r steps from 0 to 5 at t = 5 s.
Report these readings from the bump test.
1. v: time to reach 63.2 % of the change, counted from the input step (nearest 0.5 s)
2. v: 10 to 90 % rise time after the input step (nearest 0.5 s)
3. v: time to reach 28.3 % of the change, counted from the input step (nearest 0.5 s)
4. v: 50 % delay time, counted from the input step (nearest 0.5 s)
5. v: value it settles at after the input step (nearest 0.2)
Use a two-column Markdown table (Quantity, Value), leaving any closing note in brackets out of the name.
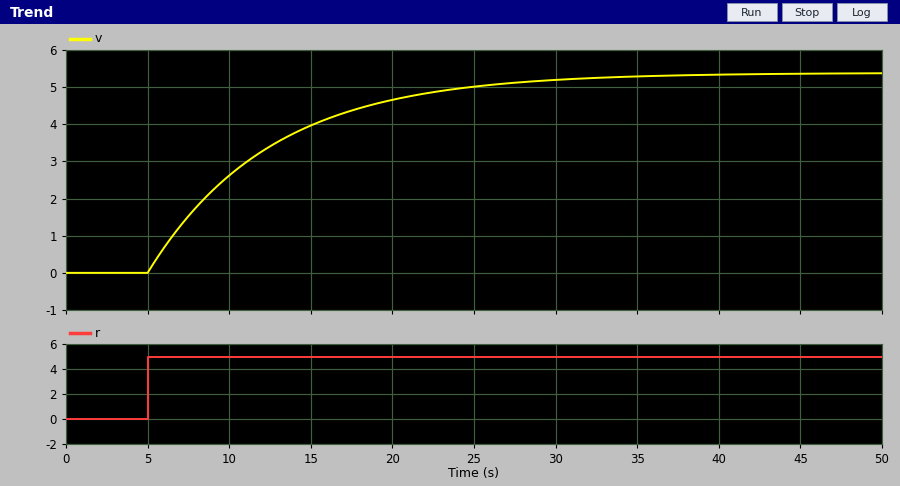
| Quantity | Value |
|---|---|
| v: time to reach 63.2 % of the change, counted from the input step | 7.5 s |
| v: 10 to 90 % rise time after the input step | 16.5 s |
| v: time to reach 28.3 % of the change, counted from the input step | 2.5 s |
| v: 50 % delay time, counted from the input step | 5.0 s |
| v: value it settles at after the input step | 5.4 |
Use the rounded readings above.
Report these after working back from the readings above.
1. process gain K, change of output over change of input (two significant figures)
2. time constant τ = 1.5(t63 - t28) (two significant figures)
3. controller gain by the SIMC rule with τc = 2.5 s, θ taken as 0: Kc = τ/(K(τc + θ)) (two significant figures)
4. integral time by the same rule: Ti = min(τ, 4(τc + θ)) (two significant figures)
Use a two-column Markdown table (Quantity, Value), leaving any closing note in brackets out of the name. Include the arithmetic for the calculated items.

| Quantity | Value |
|---|---|
| process gain K, change of output over change of input | (5.4 - 0) / 5 = 1.1 |
| time constant τ = 1.5(t63 - t28) | 1.5 × (7.5 - 2.5) = 7.5 s |
| controller gain by the SIMC rule with τc = 2.5 s, θ taken as 0: Kc = τ/(K(τc + θ)) | 7.5 / (1.1 × (2.5 + 0)) = 2.7 |
| integral time by the same rule: Ti = min(τ, 4(τc + θ)) | min(7.5, 4 × (2.5 + 0)) = 7.5 s |
